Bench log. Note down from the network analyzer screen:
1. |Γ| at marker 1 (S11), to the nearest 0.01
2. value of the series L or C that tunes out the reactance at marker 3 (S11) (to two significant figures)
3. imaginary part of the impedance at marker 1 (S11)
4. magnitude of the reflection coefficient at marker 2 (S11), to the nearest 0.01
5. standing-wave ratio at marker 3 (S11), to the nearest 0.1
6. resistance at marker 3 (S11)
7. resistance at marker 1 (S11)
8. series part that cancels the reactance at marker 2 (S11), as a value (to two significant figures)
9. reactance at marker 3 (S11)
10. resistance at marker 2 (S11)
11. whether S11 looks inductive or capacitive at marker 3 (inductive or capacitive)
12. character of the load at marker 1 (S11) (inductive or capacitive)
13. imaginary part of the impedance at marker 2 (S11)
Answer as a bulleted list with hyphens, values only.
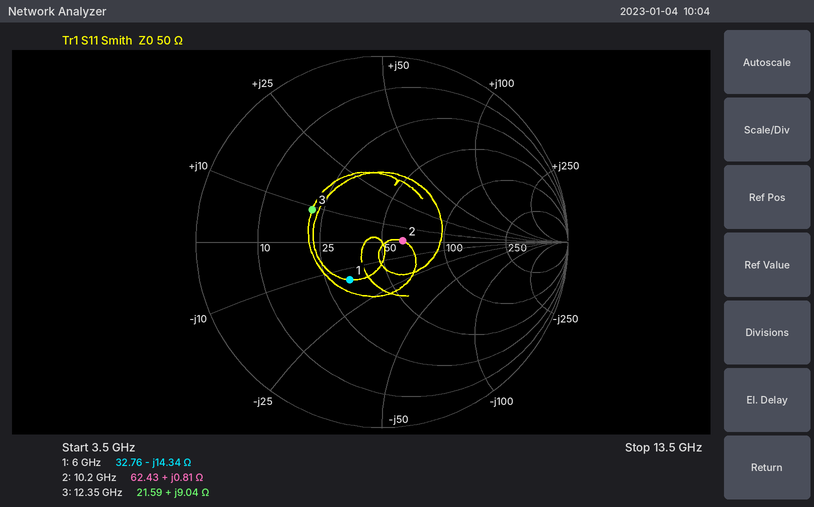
- 0.27
- 1.4 pF
- -14.34 Ω
- 0.11
- 2.4
- 21.59 Ω
- 32.76 Ω
- 19 pF
- +9.04 Ω
- 62.43 Ω
- inductive
- capacitive
- +0.81 Ω
